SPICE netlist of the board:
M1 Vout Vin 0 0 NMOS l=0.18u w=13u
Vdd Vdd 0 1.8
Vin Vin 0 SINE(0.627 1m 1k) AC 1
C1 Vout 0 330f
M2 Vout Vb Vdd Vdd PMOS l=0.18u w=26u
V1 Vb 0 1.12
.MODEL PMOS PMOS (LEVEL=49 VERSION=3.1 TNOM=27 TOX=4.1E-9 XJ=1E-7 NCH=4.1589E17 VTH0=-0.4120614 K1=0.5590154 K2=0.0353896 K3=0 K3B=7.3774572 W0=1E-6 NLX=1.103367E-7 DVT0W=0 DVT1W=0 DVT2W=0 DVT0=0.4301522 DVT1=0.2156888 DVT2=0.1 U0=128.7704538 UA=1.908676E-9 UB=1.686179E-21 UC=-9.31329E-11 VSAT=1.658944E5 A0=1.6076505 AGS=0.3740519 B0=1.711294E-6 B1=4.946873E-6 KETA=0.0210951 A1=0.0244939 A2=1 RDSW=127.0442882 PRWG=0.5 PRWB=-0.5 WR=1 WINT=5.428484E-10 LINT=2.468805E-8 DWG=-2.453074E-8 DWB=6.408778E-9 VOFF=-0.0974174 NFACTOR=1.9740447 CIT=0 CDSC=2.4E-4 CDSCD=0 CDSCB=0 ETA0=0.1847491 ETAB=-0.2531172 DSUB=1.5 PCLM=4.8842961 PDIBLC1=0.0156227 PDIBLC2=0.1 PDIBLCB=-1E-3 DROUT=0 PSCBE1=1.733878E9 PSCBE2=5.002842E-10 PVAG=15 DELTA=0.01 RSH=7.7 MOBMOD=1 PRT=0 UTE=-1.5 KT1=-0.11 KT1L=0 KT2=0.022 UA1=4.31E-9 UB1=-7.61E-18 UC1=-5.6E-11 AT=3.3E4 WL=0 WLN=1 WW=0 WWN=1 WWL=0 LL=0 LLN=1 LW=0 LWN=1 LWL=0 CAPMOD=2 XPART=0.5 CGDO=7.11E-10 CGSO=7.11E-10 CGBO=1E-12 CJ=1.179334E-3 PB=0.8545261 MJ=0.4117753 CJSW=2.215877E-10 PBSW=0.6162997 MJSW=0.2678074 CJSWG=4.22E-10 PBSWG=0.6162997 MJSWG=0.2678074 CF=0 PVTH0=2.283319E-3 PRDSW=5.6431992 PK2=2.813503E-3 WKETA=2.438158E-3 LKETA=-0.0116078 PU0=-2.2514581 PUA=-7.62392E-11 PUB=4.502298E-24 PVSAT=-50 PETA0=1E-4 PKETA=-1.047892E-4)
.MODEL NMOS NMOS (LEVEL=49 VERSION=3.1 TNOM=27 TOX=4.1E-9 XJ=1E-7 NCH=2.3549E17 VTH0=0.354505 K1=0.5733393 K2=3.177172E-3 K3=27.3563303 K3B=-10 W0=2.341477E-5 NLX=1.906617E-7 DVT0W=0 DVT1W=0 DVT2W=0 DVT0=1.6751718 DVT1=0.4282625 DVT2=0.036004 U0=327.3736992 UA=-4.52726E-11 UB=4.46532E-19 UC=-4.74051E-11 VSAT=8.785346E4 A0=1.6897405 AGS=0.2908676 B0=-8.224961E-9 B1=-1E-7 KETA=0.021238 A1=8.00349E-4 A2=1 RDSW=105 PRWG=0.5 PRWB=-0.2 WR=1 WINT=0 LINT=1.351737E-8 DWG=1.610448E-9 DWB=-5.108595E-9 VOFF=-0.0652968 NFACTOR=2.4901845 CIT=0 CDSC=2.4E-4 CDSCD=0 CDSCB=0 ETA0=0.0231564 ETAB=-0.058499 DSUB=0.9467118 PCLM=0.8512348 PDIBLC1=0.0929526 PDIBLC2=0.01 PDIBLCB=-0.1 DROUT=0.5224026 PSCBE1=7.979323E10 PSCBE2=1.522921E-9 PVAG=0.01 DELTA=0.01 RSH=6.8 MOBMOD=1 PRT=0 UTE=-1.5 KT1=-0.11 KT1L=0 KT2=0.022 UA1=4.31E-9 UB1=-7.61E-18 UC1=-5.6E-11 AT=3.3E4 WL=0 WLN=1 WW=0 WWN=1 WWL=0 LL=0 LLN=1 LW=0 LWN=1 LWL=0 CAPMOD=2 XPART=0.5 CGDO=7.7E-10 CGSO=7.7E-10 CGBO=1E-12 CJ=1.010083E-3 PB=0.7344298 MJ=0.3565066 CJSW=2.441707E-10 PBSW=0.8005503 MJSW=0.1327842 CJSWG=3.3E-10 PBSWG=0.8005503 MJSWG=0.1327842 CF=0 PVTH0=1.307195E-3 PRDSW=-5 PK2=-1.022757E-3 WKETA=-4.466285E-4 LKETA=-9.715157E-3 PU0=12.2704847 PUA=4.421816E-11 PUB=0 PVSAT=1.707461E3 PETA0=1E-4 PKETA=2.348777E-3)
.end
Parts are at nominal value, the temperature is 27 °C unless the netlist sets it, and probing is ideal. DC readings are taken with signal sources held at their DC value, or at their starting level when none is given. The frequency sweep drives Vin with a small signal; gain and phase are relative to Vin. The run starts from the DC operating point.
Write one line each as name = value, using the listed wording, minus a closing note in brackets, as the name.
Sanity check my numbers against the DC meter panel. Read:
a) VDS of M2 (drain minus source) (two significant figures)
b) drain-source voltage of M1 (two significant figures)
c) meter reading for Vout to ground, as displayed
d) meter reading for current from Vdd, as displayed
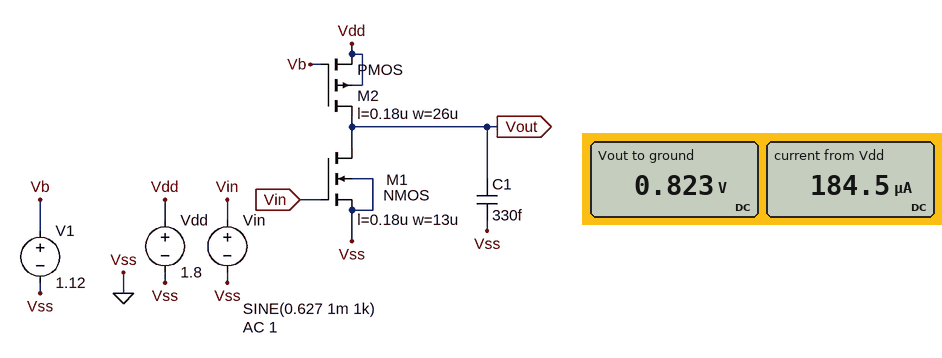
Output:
VDS of M2 (drain minus source) = -980 mV
drain-source voltage of M1 = 820 mV
meter reading for Vout to ground, as displayed = 0.823 V
meter reading for current from Vdd, as displayed = 184.5 µA
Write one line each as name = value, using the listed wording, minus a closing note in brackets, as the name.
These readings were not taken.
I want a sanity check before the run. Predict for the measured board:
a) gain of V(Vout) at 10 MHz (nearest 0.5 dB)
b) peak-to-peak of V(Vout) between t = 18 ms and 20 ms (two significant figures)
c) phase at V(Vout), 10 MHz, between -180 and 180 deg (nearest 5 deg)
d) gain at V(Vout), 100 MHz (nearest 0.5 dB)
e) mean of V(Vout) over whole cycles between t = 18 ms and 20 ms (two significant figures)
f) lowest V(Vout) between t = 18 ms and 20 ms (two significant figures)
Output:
gain of V(Vout) at 10 MHz = 28.0 dB
peak-to-peak of V(Vout) between t = 18 ms and 20 ms = 53 mV
phase at V(Vout), 10 MHz, between -180 and 180 deg = 165 deg
gain at V(Vout), 100 MHz = 20.0 dB
mean of V(Vout) over whole cycles between t = 18 ms and 20 ms = 820 mV
lowest V(Vout) between t = 18 ms and 20 ms = 800 mV
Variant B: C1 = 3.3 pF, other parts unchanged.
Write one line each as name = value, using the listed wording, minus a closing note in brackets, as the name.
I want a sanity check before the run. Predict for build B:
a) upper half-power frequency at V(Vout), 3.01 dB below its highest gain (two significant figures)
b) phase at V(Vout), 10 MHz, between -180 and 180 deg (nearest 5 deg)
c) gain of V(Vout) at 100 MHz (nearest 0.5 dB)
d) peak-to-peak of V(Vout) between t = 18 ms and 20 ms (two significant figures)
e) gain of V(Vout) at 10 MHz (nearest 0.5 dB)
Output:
upper half-power frequency at V(Vout), 3.01 dB below its highest gain = 4.6 MHz
phase at V(Vout), 10 MHz, between -180 and 180 deg = 115 deg
gain of V(Vout) at 100 MHz = 1.5 dB
peak-to-peak of V(Vout) between t = 18 ms and 20 ms = 53 mV
gain of V(Vout) at 10 MHz = 21.0 dB
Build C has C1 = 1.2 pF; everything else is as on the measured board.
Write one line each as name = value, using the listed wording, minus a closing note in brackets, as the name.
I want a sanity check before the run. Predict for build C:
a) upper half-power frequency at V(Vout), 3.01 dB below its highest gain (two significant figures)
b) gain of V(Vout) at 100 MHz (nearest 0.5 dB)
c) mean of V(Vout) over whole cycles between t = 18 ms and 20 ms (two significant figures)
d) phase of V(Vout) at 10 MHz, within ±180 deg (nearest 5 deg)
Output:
upper half-power frequency at V(Vout), 3.01 dB below its highest gain = 12 MHz
gain of V(Vout) at 100 MHz = 10.0 dB
mean of V(Vout) over whole cycles between t = 18 ms and 20 ms = 820 mV
phase of V(Vout) at 10 MHz, within ±180 deg = 140 deg
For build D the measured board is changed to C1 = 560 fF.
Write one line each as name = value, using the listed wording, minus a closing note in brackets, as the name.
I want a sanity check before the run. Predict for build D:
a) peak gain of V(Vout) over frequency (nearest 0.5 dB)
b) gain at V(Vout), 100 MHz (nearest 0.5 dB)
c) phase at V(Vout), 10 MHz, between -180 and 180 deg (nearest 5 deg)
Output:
peak gain of V(Vout) over frequency = 28.5 dB
gain at V(Vout), 100 MHz = 16.5 dB
phase at V(Vout), 10 MHz, between -180 and 180 deg = 160 deg
